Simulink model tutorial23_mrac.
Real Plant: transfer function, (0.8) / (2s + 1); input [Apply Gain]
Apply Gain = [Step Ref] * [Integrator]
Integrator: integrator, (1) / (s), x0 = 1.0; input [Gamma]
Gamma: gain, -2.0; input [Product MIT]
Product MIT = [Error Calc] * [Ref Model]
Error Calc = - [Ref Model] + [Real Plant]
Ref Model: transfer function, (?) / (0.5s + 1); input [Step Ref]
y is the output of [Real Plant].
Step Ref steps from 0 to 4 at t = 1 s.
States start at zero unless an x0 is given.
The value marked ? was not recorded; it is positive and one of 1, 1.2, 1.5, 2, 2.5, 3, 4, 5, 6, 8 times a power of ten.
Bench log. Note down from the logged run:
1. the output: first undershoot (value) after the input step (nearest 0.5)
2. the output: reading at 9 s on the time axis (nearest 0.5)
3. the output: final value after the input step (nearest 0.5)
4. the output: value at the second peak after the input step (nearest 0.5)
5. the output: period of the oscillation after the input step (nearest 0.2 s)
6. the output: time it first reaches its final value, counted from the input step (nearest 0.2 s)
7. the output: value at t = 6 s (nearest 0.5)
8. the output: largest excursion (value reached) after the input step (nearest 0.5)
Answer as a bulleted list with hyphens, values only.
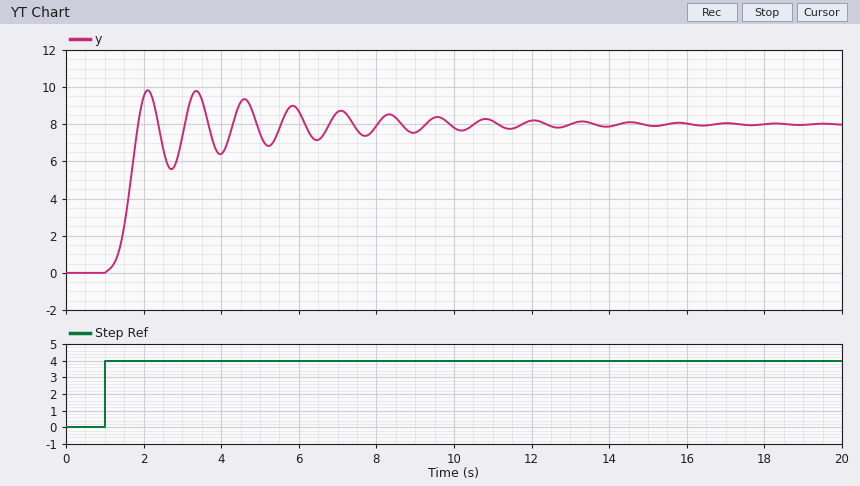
- 5.5
- 7.5
- 8.0
- 10.0
- 1.2 s
- 0.8 s
- 8.5
- 10.0
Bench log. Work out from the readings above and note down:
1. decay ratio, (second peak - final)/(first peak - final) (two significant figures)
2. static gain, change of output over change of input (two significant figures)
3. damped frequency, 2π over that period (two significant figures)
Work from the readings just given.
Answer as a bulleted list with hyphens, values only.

- 1.0
- 2.0
- 5.2 rad/s
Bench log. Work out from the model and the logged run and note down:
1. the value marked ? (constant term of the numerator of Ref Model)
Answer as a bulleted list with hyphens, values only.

- 2
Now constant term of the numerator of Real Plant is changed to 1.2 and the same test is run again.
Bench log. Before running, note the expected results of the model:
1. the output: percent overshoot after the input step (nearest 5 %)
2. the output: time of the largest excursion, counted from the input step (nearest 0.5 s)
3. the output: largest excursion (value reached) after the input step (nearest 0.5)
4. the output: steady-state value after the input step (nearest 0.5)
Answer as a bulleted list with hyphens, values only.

- 20 %
- 2.0 s
- 9.5
- 8.0
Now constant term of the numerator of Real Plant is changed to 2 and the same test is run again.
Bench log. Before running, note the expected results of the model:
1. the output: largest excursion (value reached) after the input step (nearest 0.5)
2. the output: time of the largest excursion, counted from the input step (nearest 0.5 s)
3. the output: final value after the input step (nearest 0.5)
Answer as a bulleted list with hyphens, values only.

- 9.0
- 1.5 s
- 8.0
